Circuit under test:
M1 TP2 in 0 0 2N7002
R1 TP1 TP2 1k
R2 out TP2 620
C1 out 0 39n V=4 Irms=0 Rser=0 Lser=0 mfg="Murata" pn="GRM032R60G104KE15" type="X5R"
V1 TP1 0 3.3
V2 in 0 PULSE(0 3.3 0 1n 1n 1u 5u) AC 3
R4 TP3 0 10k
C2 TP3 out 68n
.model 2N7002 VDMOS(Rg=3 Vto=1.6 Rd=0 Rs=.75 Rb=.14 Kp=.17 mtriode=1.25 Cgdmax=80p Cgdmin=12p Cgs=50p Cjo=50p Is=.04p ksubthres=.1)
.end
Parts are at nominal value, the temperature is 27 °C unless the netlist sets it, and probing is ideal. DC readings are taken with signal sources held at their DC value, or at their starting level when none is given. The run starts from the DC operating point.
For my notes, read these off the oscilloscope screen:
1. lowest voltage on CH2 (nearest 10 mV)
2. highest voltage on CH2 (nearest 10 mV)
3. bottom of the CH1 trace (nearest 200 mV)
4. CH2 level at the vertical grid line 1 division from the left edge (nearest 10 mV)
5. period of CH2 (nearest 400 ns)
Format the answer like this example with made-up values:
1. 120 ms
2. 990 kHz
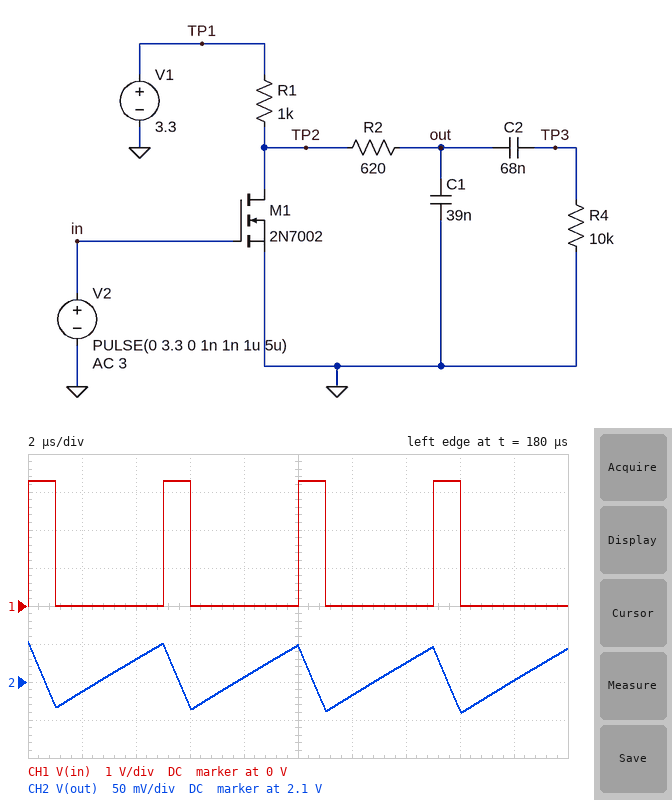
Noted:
1. 2.06 V
2. 2.15 V
3. 0 V
4. 2.09 V
5. 5.2 µs
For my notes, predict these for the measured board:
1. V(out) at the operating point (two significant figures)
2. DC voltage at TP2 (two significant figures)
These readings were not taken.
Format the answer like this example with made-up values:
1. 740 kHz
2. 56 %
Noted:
1. 3.3 V
2. 3.3 V
